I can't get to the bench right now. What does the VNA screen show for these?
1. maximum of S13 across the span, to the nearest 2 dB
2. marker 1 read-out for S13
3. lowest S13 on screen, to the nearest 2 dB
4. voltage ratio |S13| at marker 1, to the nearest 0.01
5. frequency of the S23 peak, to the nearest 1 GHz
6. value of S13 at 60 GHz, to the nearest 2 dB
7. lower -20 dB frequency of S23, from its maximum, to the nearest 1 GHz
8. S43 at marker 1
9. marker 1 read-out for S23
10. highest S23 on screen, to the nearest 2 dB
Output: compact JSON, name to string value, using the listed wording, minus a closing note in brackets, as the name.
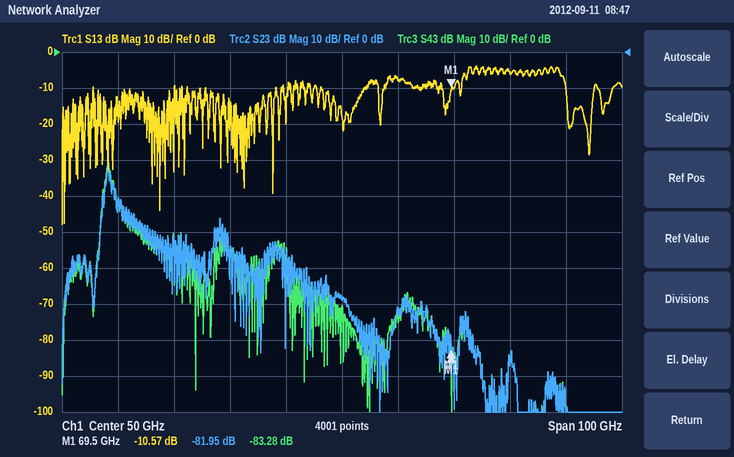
{"maximum of S13 across the span, to the nearest 2 dB": "-4 dB", "marker 1 read-out for S13": "-10.57 dB", "lowest S13 on screen, to the nearest 2 dB": "-48 dB", "voltage ratio |S13| at marker 1, to the nearest 0.01": "0.30", "frequency of the S23 peak, to the nearest 1 GHz": "8 GHz", "value of S13 at 60 GHz, to the nearest 2 dB": "-8 dB", "lower -20 dB frequency of S23, from its maximum, to the nearest 1 GHz": "7 GHz", "S43 at marker 1": "-83.28 dB", "marker 1 read-out for S23": "-81.95 dB", "highest S23 on screen, to the nearest 2 dB": "-32 dB"}
